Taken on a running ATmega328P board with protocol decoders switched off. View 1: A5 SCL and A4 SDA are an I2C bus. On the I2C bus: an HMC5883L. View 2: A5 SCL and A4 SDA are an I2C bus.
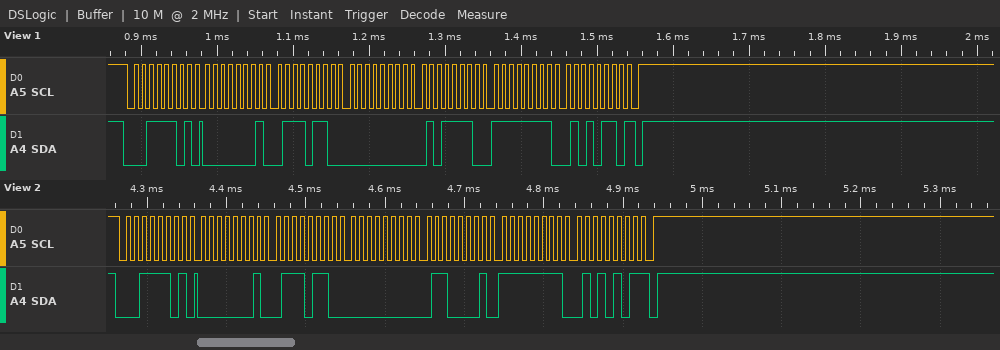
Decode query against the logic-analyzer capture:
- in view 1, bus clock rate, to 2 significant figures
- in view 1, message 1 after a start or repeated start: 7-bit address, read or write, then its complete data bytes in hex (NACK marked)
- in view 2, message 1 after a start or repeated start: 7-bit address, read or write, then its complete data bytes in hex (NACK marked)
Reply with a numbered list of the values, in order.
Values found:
1. 100 kHz
2. 0x1E read: 01 76 00 5E FF 56 NACK
3. 0x1E read: 01 76 00 61 FF 55 NACK
